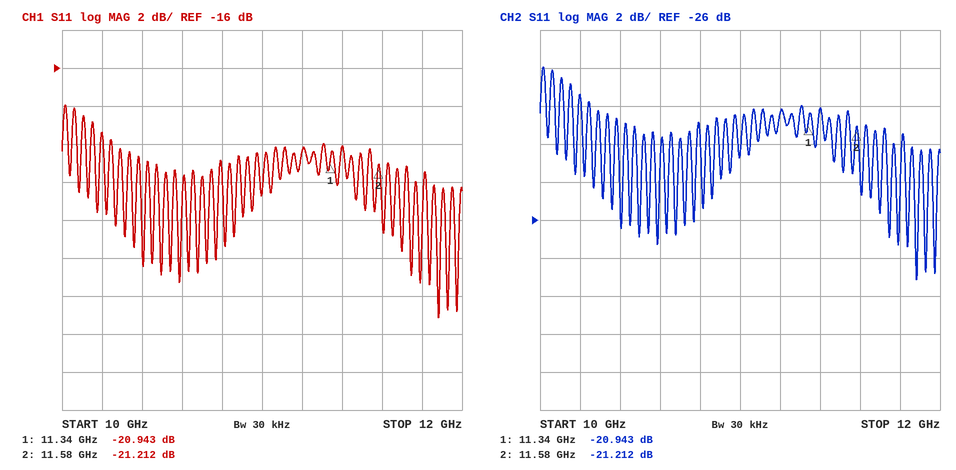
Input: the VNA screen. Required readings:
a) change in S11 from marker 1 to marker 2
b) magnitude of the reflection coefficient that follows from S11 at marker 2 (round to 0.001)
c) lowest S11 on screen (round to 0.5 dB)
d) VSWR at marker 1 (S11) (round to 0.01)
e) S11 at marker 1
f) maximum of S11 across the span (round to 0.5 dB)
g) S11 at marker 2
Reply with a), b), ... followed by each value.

a) -0.269 dB
b) 0.087
c) -29.0 dB
d) 1.20
e) -20.943 dB
f) -18.0 dB
g) -21.212 dB
